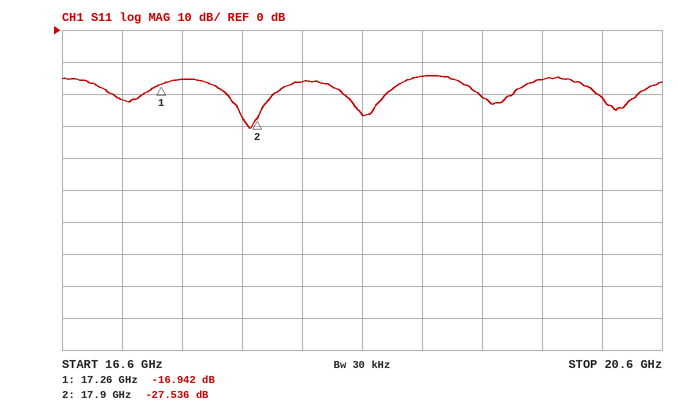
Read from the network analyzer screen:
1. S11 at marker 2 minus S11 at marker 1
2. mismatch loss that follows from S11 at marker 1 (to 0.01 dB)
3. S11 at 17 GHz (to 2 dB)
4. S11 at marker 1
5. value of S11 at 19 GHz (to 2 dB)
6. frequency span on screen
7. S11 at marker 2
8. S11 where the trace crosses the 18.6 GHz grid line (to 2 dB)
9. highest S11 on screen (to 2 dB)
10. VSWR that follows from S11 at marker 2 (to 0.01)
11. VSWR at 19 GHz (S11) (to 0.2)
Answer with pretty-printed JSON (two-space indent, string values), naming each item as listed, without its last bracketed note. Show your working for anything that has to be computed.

{
  "S11 at marker 2 minus S11 at marker 1": "-27.536 − (-16.942) = -10.594 dB",
  "mismatch loss that follows from S11 at marker 1": "−10 log10(1 − 10^(-16.942/10)) ≈ 0.09 dB",
  "S11 at 17 GHz": "-22 dB",
  "S11 at marker 1": "-16.942 dB",
  "value of S11 at 19 GHz": "-14 dB",
  "frequency span on screen": "4 GHz",
  "S11 at marker 2": "-27.536 dB",
  "S11 where the trace crosses the 18.6 GHz grid line": "-26 dB",
  "highest S11 on screen": "-14 dB",
  "VSWR that follows from S11 at marker 2": "(1 + 0.0420)/(1 − 0.0420) ≈ 1.09",
  "VSWR at 19 GHz (S11)": "|Γ| = 10^(-14/20) = 0.1995; VSWR = (1 + 0.1995)/(1 − 0.1995) ≈ 1.50, so 1.4 to the nearest 0.2"
}
